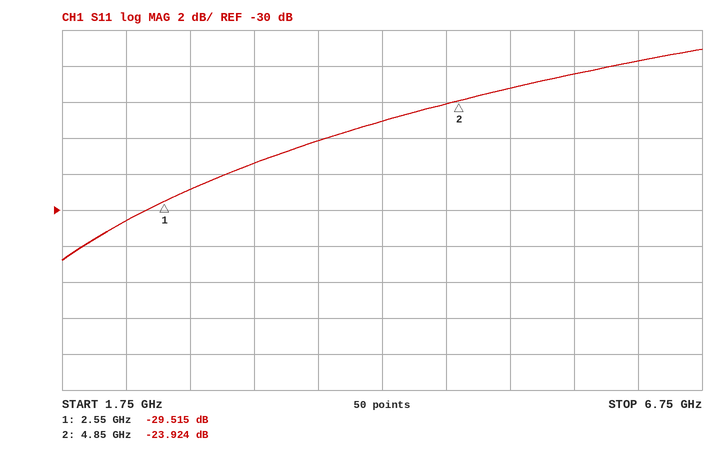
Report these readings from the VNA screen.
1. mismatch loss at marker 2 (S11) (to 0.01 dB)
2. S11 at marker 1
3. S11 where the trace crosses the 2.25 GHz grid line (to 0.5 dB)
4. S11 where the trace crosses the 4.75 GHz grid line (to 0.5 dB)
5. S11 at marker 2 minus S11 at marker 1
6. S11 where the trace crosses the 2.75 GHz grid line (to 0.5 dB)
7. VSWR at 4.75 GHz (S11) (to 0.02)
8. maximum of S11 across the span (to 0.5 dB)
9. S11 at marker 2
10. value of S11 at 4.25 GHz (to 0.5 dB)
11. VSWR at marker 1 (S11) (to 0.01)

0.02 dB
-29.515 dB
-30.5 dB
-24.0 dB
5.591 dB
-29.0 dB
1.14
-21.0 dB
-23.924 dB
-25.0 dB
1.07
